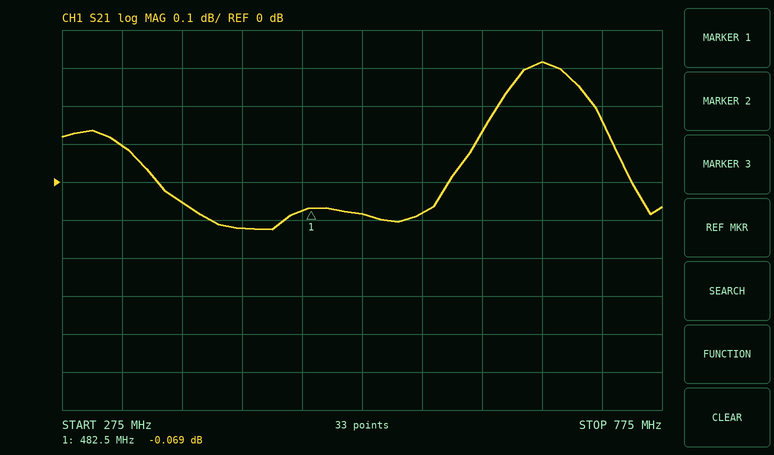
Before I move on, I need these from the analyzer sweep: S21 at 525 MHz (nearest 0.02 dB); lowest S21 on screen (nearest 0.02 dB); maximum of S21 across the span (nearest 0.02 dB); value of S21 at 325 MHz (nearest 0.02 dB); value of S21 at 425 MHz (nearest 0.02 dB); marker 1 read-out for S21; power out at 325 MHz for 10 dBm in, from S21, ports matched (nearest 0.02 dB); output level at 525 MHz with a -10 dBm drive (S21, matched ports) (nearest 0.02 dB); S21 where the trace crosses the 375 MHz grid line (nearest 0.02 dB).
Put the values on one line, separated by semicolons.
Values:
-0.08 dB; -0.12 dB; 0.32 dB; 0.10 dB; -0.12 dB; -0.069 dB; 10.10 dBm; -10.08 dBm; -0.06 dB
